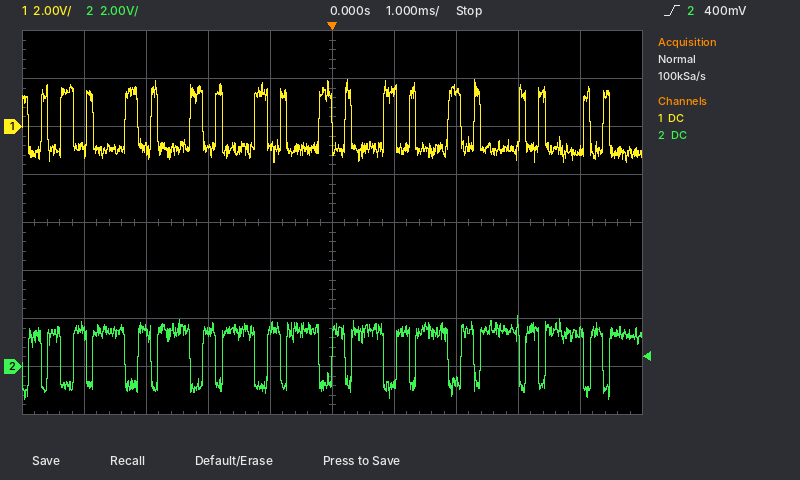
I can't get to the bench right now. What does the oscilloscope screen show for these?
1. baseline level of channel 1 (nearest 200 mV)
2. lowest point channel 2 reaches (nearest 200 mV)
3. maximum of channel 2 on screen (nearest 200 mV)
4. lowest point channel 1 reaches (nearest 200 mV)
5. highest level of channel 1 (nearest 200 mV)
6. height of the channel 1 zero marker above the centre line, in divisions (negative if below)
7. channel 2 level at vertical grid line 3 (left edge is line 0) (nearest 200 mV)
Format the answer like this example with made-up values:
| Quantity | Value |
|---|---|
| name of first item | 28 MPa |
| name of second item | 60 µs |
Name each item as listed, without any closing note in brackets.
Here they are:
| Quantity | Value |
|---|---|
| baseline level of channel 1 | -1.0 V |
| lowest point channel 2 reaches | -1.4 V |
| maximum of channel 2 on screen | 2.2 V |
| lowest point channel 1 reaches | -1.6 V |
| highest level of channel 1 | 2.0 V |
| height of the channel 1 zero marker above the centre line, in divisions | +2.0 div |
| channel 2 level at vertical grid line 3 (left edge is line 0) | 1.4 V |
